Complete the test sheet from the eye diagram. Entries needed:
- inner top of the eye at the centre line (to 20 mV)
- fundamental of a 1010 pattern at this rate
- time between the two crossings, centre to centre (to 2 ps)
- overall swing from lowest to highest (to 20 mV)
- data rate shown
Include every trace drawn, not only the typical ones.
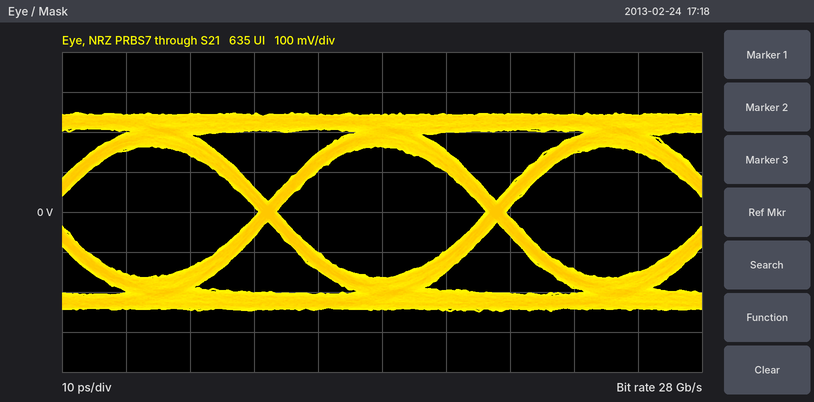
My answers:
160 mV
14 GHz
36 ps
500 mV
28 Gb/s
